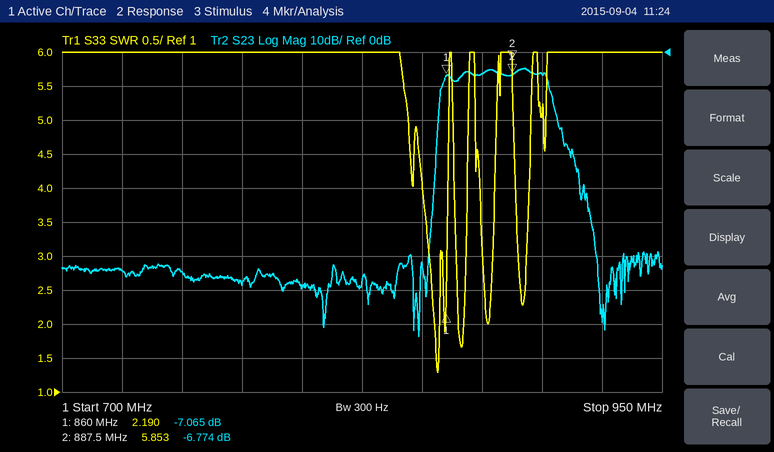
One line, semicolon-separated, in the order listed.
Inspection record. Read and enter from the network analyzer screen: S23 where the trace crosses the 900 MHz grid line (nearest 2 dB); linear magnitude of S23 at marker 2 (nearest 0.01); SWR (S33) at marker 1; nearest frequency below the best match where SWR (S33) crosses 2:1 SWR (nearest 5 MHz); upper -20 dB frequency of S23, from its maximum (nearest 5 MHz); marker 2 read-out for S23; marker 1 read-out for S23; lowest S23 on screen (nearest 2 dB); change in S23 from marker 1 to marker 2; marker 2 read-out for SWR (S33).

-6 dB; 0.46; 2.190; 855 MHz; 910 MHz; -6.774 dB; -7.065 dB; -84 dB; 0.291 dB; 5.853
